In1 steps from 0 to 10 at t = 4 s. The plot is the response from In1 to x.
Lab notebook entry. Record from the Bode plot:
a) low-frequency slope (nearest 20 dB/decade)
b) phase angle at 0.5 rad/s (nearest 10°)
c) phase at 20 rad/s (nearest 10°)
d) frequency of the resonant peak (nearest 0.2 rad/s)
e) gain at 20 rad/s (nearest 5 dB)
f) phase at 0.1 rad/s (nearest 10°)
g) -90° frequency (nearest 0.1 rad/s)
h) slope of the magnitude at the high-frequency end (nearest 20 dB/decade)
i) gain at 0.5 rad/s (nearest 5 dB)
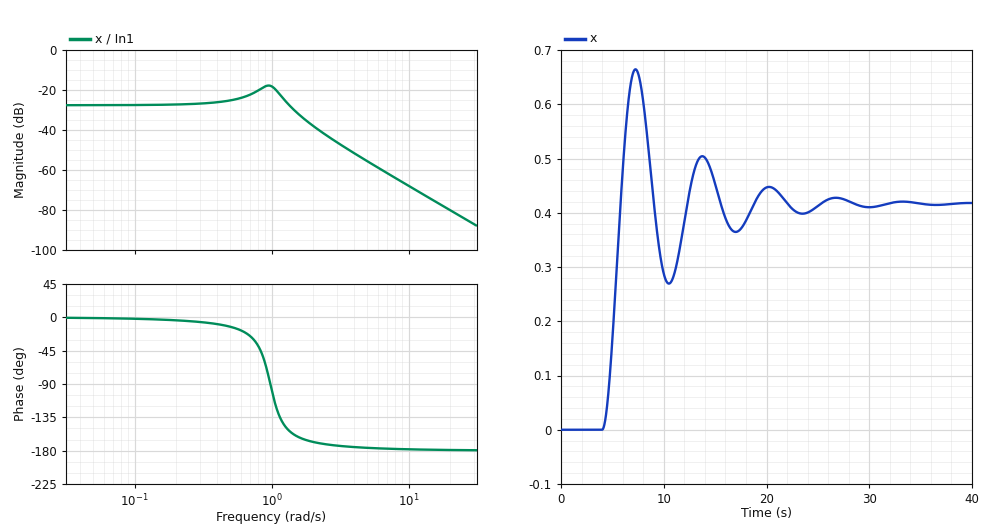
0 dB/decade
-10°
-180°
1.0 rad/s
-80 dB
0°
1.0 rad/s
-40 dB/decade
-25 dB
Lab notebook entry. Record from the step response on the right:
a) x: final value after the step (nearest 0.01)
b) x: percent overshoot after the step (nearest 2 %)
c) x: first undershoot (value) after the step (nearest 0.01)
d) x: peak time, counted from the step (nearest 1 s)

0.42
60 %
0.27
3 s
